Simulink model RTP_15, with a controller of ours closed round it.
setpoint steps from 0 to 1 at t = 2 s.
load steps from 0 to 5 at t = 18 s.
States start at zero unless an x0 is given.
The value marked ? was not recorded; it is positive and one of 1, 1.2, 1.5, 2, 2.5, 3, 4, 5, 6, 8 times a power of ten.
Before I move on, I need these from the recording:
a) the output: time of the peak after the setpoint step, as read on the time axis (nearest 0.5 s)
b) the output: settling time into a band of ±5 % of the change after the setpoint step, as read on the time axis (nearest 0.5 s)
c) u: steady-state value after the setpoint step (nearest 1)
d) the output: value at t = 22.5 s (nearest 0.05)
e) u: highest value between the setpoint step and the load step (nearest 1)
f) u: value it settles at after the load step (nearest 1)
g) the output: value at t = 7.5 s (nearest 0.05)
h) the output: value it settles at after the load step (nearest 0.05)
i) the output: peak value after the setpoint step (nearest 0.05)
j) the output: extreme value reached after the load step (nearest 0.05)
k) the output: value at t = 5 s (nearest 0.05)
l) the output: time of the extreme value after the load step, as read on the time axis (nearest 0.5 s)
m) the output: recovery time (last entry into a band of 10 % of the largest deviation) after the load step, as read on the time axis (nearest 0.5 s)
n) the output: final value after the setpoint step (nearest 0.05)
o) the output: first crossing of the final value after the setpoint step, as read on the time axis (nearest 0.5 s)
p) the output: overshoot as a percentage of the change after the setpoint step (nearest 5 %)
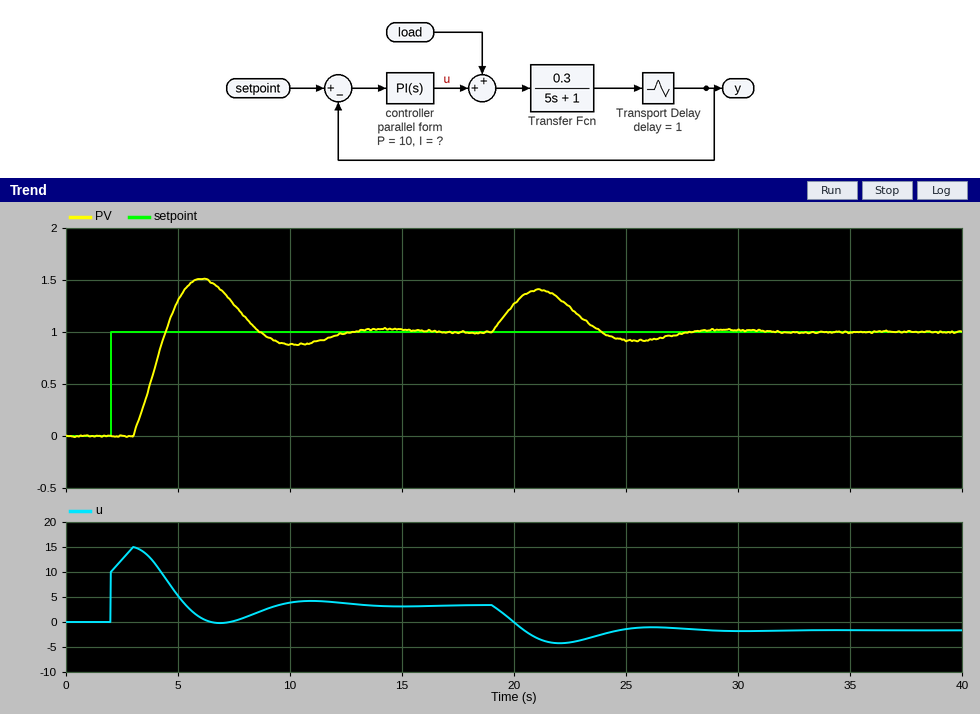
6.0 s
12.0 s
3
1.25
15
-2
1.25
1.00
1.50
1.40
1.30
21.0 s
27.0 s
1.00
4.5 s
50 %
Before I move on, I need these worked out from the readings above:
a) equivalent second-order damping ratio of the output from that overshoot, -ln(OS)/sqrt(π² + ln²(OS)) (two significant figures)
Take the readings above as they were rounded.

0.22
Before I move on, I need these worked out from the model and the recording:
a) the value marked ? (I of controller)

5
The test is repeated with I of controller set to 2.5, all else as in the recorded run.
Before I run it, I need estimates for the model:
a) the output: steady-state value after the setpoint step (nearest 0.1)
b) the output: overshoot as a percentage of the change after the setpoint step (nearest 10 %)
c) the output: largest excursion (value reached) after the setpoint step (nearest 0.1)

1.0
20 %
1.2
